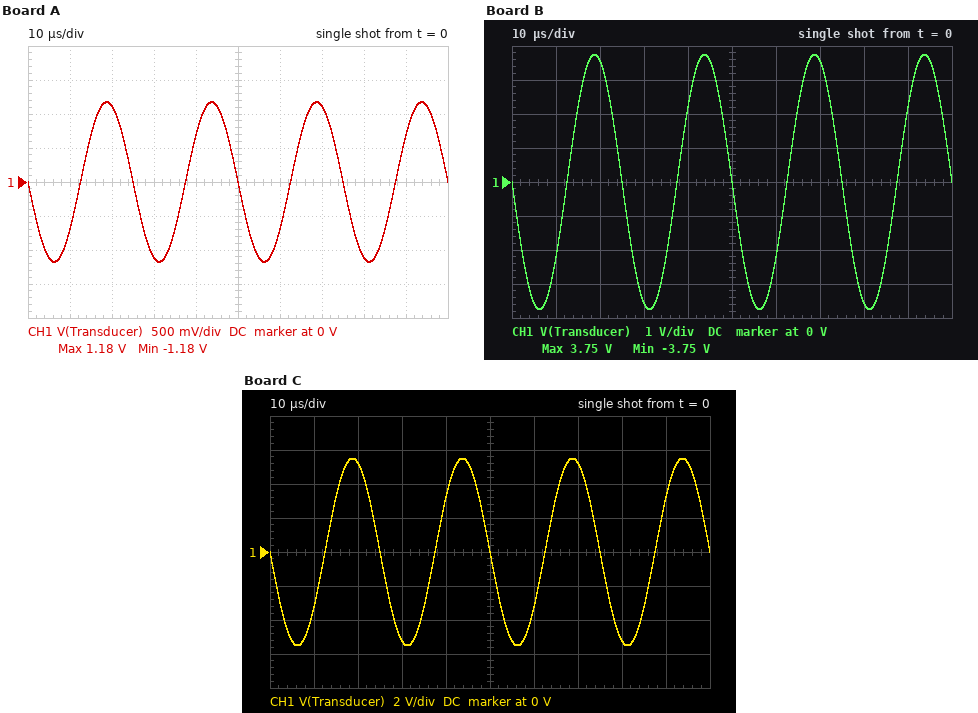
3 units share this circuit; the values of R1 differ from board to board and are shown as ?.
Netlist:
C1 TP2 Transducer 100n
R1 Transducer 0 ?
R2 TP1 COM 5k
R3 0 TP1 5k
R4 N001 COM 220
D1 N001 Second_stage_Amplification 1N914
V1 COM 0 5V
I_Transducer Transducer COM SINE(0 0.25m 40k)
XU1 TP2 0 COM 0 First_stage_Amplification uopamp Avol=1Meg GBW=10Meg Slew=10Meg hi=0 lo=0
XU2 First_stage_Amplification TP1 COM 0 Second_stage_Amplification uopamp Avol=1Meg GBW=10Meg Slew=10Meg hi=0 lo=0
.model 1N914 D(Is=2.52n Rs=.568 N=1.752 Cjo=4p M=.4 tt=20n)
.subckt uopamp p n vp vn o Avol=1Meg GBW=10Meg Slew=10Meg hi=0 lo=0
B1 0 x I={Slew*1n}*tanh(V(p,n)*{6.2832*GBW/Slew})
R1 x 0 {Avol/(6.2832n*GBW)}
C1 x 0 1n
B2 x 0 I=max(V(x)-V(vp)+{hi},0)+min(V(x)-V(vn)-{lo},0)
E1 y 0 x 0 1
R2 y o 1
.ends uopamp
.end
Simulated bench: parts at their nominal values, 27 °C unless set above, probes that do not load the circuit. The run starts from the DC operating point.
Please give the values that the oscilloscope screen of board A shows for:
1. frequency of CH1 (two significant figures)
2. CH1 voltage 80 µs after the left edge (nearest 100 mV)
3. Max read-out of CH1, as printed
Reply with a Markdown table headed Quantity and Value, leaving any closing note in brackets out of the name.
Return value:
| Quantity | Value |
|---|---|
| frequency of CH1 | 40 kHz |
| CH1 voltage 80 µs after the left edge | -1.1 V |
| Max read-out of CH1, as printed | 1.18 V |
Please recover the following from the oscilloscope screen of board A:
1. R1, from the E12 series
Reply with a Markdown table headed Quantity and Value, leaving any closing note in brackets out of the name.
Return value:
| Quantity | Value |
|---|---|
| R1, from the E12 series | 4.7 kΩ |
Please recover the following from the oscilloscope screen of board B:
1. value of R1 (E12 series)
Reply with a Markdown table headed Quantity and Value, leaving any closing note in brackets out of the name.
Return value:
| Quantity | Value |
|---|---|
| value of R1 | 15 kΩ |
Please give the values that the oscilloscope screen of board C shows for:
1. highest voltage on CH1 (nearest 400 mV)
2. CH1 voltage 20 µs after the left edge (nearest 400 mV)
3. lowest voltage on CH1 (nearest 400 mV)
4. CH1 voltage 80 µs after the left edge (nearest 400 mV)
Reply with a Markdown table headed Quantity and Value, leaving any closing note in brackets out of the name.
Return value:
| Quantity | Value |
|---|---|
| highest voltage on CH1 | 5.6 V |
| CH1 voltage 20 µs after the left edge | 5.2 V |
| lowest voltage on CH1 | -5.6 V |
| CH1 voltage 80 µs after the left edge | -5.2 V |
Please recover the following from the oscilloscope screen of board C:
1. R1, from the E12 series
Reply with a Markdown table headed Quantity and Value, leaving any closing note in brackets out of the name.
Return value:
| Quantity | Value |
|---|---|
| R1, from the E12 series | 22 kΩ |
